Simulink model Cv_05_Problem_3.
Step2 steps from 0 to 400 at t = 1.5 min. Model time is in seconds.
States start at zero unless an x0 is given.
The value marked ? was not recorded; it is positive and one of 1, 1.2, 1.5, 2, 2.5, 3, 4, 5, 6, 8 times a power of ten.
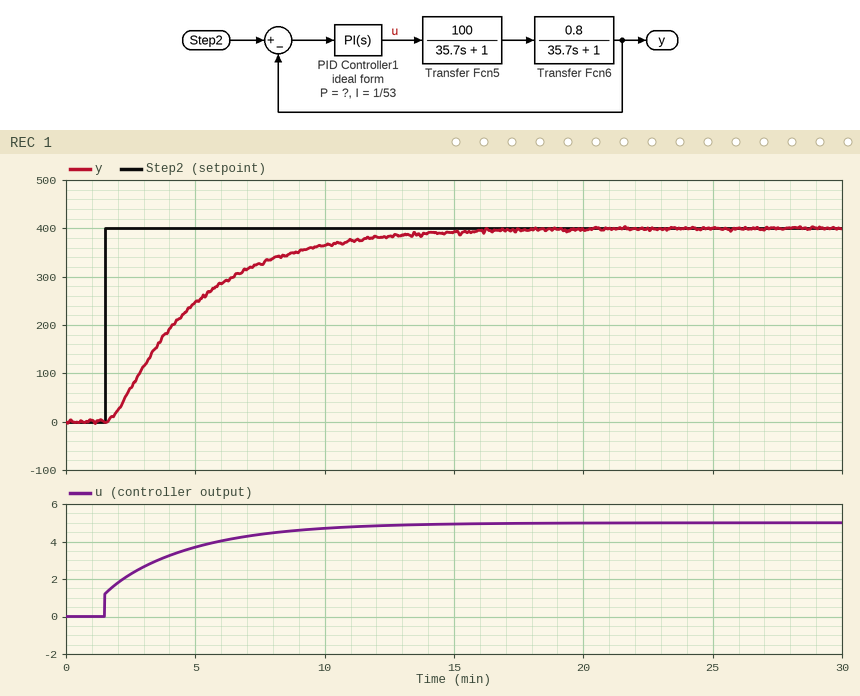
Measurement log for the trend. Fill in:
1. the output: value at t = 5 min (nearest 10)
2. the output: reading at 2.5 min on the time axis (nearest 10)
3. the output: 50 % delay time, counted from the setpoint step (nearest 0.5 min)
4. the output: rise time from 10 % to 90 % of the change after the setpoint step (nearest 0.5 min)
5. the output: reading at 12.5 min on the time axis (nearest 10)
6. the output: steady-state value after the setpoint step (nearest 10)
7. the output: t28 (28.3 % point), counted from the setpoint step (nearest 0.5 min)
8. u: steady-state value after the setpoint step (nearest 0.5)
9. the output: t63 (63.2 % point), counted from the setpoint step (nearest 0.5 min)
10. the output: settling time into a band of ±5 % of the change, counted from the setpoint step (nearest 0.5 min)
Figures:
250
70
2.5 min
7.5 min
380
400
1.5 min
5.0
3.5 min
10.5 min
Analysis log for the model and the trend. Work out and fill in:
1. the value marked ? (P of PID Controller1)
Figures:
0.003
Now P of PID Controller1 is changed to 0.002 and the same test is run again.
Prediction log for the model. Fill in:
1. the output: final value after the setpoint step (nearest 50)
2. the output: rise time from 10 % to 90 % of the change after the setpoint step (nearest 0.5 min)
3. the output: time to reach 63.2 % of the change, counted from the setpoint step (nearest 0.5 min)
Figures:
400
11.5 min
5.5 min
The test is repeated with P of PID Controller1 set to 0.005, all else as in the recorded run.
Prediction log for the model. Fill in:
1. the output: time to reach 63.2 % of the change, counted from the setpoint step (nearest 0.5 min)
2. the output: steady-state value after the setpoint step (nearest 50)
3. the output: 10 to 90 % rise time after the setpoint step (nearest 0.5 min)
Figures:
2.0 min
400
4.0 min
